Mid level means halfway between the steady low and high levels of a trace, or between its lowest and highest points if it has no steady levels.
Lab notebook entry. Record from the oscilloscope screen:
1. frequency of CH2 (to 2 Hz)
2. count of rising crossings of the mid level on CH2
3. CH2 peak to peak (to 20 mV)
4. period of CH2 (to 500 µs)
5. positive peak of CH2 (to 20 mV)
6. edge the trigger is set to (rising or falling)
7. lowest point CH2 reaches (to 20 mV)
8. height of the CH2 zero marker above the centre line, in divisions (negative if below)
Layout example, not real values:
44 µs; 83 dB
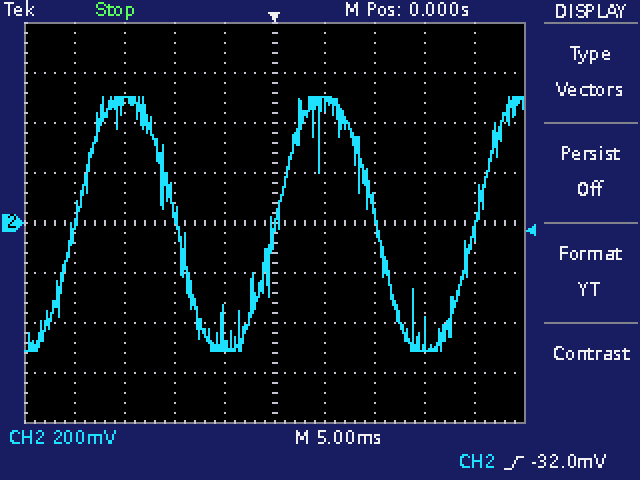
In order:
50 Hz; 3; 1.02 V; 20.0 ms; 500 mV; rising; -520 mV; 0.0 div
